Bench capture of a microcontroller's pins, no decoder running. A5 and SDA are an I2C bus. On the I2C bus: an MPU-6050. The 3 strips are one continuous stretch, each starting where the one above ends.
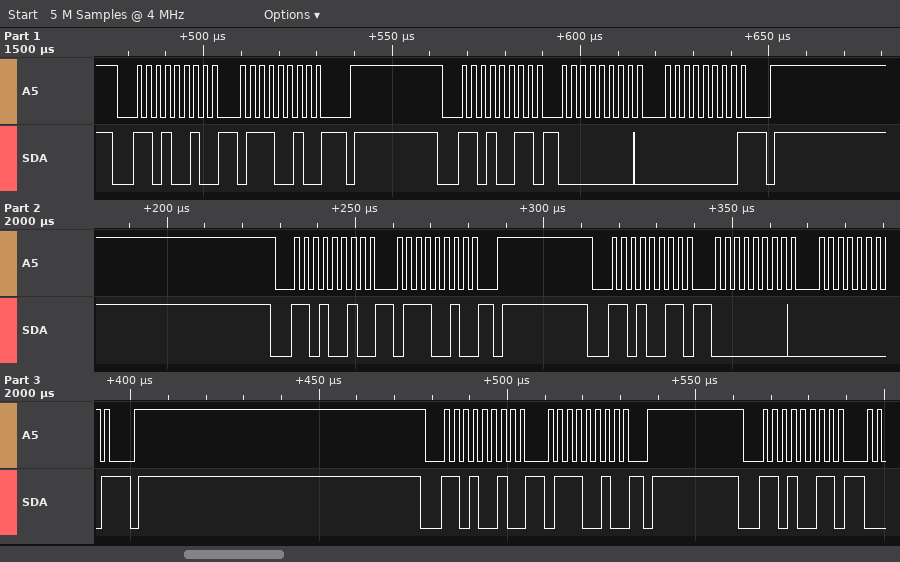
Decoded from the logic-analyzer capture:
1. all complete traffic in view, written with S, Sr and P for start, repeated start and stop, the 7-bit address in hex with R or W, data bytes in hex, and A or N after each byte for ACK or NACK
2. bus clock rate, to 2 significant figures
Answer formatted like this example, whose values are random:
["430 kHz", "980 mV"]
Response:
["S 69W A 72 A P S 69R A 00 A 00 N P S 69W A 72 A P S 69R A 00 A 00 N P S 69W A 72 A P S 69R A", "400 kHz"]
